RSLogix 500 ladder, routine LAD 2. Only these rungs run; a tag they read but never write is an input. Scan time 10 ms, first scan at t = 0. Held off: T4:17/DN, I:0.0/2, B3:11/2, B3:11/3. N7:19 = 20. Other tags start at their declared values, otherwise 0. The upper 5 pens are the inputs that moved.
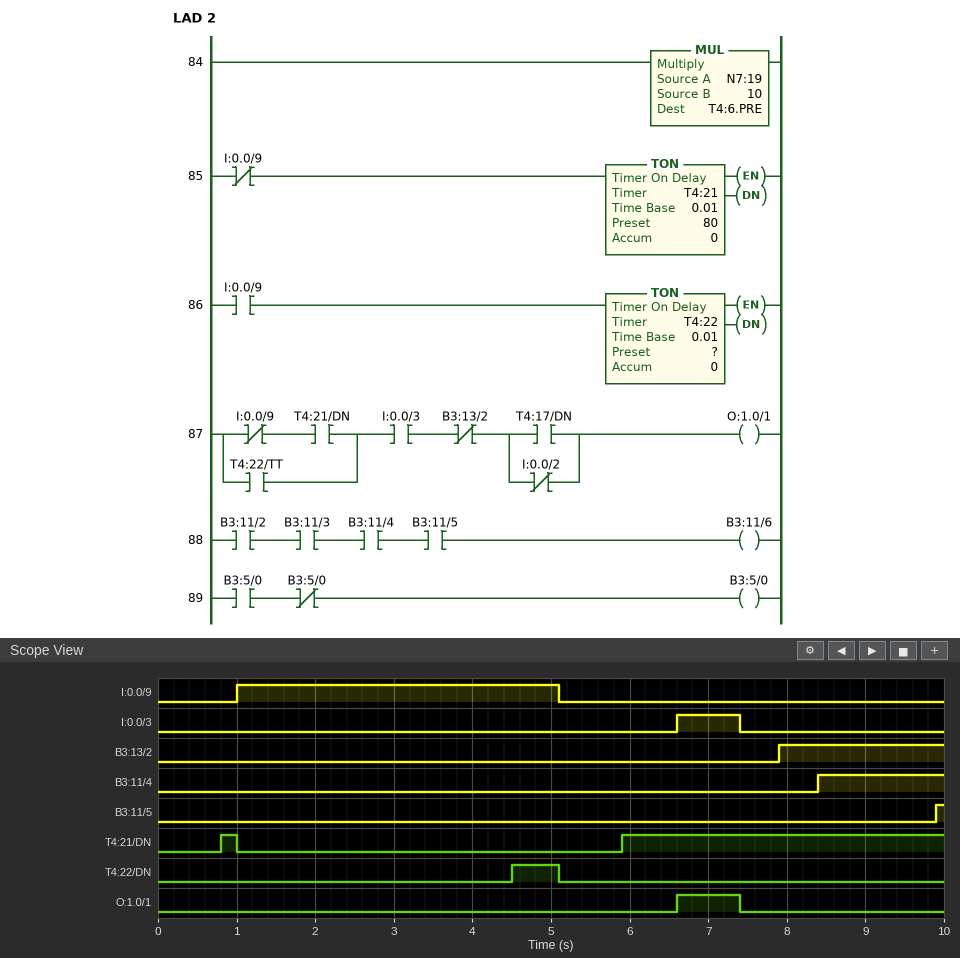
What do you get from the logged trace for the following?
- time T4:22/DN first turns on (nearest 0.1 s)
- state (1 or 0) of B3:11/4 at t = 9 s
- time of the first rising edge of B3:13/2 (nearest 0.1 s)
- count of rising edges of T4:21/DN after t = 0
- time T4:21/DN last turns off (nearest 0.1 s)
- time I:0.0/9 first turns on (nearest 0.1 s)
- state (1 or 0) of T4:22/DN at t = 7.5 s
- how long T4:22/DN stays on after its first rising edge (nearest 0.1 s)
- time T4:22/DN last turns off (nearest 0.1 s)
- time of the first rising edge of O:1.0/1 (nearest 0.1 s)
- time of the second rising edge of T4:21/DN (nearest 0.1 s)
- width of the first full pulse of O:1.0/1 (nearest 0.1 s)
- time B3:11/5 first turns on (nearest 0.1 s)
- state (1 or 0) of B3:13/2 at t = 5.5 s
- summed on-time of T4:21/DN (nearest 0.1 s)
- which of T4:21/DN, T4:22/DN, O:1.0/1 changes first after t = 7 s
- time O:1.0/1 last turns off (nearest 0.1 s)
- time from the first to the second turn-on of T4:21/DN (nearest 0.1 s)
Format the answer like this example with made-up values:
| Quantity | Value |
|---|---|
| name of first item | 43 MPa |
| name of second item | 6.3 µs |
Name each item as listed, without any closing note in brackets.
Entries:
| Quantity | Value |
|---|---|
| time T4:22/DN first turns on | 4.5 s |
| state (1 or 0) of B3:11/4 at t = 9 s | 1 |
| time of the first rising edge of B3:13/2 | 7.9 s |
| count of rising edges of T4:21/DN after t = 0 | 2 |
| time T4:21/DN last turns off | 1.0 s |
| time I:0.0/9 first turns on | 1.0 s |
| state (1 or 0) of T4:22/DN at t = 7.5 s | 0 |
| how long T4:22/DN stays on after its first rising edge | 0.6 s |
| time T4:22/DN last turns off | 5.1 s |
| time of the first rising edge of O:1.0/1 | 6.6 s |
| time of the second rising edge of T4:21/DN | 5.9 s |
| width of the first full pulse of O:1.0/1 | 0.8 s |
| time B3:11/5 first turns on | 9.9 s |
| state (1 or 0) of B3:13/2 at t = 5.5 s | 0 |
| summed on-time of T4:21/DN | 4.3 s |
| which of T4:21/DN, T4:22/DN, O:1.0/1 changes first after t = 7 s | O:1.0/1 |
| time O:1.0/1 last turns off | 7.4 s |
| time from the first to the second turn-on of T4:21/DN | 5.1 s |
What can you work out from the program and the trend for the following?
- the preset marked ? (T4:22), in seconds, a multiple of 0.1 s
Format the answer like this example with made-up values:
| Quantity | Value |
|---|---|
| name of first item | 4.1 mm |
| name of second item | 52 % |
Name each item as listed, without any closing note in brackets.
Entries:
| Quantity | Value |
|---|---|
| the preset marked ? (T4:22), in seconds, a multiple of 0.1 s | 3.5 s |
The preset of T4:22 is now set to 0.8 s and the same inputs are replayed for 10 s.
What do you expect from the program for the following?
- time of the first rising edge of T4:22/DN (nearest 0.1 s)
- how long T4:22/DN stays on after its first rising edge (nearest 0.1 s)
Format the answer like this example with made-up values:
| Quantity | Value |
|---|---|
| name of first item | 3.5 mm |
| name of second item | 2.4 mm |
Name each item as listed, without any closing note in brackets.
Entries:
| Quantity | Value |
|---|---|
| time of the first rising edge of T4:22/DN | 1.8 s |
| how long T4:22/DN stays on after its first rising edge | 3.3 s |
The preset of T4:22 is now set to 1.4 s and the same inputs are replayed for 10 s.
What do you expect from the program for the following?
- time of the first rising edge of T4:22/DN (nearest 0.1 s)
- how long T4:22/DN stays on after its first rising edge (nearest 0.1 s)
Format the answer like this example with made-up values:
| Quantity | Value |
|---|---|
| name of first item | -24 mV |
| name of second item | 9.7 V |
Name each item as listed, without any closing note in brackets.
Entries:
| Quantity | Value |
|---|---|
| time of the first rising edge of T4:22/DN | 2.4 s |
| how long T4:22/DN stays on after its first rising edge | 2.7 s |
